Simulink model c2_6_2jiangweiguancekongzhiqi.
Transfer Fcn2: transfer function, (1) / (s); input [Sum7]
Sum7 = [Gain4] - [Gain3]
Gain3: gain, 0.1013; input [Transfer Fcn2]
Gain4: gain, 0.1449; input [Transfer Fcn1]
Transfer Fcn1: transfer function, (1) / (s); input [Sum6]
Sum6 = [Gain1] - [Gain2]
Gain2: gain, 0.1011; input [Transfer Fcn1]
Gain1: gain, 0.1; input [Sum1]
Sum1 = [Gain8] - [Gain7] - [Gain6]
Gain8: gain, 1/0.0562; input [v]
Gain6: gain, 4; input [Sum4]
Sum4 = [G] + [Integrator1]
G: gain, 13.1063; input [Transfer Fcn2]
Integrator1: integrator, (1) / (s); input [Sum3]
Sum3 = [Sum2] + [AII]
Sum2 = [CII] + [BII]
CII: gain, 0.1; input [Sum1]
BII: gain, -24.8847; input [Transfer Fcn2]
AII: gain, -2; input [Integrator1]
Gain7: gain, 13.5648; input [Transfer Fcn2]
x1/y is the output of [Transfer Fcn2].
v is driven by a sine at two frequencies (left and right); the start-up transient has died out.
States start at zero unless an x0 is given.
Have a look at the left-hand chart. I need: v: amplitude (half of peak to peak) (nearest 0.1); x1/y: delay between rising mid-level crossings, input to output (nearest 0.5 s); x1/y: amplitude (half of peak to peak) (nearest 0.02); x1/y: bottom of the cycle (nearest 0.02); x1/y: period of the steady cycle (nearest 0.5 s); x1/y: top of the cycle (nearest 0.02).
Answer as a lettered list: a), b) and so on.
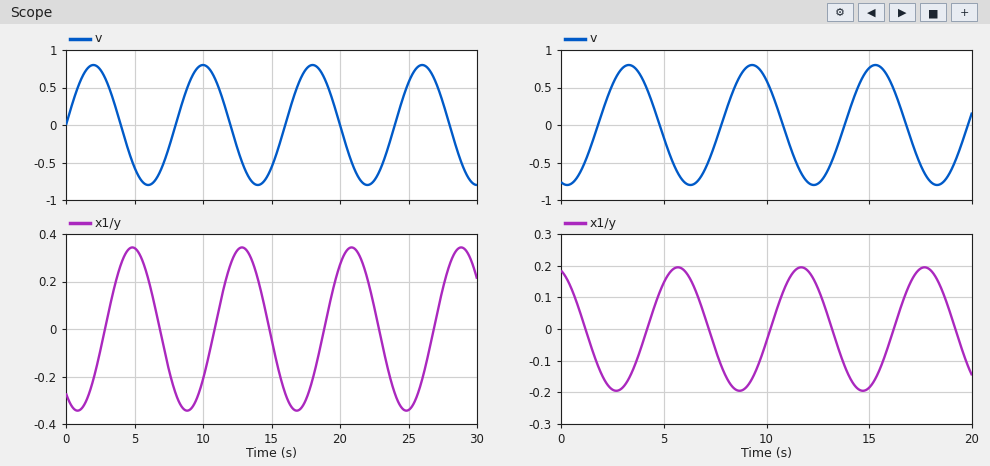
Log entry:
a) 0.8
b) 3.0 s
c) 0.34
d) -0.34
e) 8.0 s
f) 0.34
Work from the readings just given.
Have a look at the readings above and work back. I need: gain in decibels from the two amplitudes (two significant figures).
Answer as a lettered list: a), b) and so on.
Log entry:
a) -7.4 dB
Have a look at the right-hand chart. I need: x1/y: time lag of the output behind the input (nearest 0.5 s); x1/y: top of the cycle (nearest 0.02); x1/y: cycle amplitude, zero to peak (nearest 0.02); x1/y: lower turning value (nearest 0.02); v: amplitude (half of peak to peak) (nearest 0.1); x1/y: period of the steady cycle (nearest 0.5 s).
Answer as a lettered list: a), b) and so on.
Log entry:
a) 2.5 s
b) 0.20
c) 0.20
d) -0.20
e) 0.8
f) 6.0 s
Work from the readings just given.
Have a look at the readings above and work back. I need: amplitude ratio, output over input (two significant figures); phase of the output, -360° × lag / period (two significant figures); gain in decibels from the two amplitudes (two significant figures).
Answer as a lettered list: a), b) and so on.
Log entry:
a) 0.25
b) -150°
c) -12 dB
